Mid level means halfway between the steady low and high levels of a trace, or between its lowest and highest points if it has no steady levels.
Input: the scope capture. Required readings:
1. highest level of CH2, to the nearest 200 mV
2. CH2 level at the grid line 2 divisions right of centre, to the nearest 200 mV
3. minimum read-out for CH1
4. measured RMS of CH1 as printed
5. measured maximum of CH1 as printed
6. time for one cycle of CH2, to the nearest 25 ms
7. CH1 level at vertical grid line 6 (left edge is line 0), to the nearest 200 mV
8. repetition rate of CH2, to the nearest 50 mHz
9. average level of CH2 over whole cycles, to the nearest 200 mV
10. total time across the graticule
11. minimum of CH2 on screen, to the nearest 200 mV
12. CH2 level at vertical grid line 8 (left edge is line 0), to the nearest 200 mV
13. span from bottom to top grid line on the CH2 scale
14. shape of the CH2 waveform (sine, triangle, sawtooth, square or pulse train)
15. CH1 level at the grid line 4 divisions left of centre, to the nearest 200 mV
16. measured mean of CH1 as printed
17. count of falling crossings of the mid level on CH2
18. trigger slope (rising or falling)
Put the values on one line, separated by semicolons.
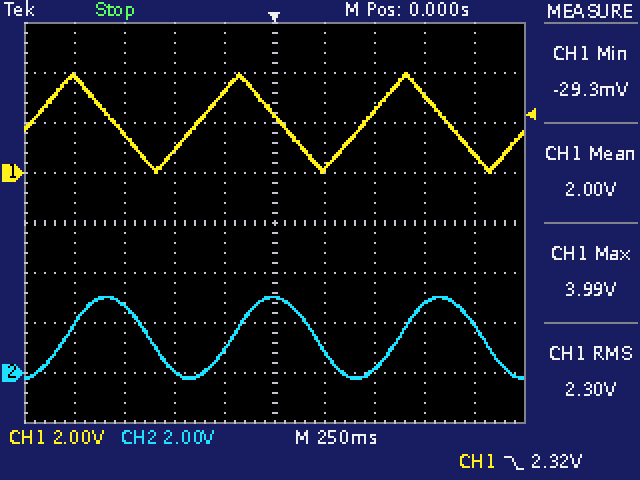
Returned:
3.0 V; 200 mV; -29.3 mV; 2.30 V; 3.99 V; 825 ms; 200 mV; 1.20 Hz; 1.4 V; 2.5 s; -200 mV; 2.8 V; 16 V; sine; 3.8 V; 2.00 V; 3; falling
